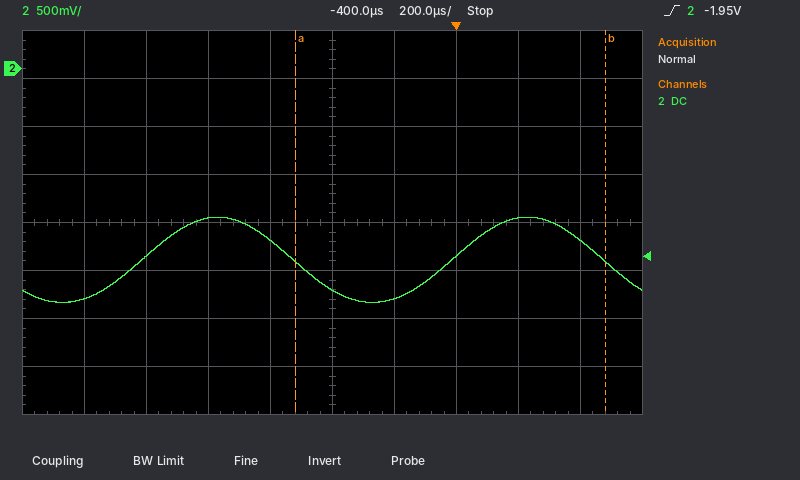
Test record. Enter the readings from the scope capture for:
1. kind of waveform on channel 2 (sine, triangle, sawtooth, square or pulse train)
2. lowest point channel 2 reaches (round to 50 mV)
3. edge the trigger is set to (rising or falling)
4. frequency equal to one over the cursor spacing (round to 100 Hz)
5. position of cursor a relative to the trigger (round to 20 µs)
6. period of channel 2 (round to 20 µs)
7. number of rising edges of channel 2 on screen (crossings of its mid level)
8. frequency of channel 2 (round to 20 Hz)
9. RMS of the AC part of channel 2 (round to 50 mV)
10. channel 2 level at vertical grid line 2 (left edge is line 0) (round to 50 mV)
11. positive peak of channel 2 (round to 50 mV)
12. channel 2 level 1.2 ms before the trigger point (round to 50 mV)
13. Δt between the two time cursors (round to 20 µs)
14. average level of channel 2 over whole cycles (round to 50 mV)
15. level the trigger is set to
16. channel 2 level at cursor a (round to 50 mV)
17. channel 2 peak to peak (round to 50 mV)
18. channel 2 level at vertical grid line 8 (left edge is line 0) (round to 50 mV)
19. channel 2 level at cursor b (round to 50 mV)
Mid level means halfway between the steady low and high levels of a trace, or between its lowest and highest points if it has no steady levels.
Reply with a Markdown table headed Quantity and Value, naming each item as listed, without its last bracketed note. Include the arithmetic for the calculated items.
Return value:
| Quantity | Value |
|---|---|
| kind of waveform on channel 2 | sine |
| lowest point channel 2 reaches | -2.45 V |
| edge the trigger is set to | rising |
| frequency equal to one over the cursor spacing | 1 / 1.00 ms ≈ 1.0 kHz |
| position of cursor a relative to the trigger | -520 µs |
| period of channel 2 | 1.00 ms |
| number of rising edges of channel 2 on screen | 2 |
| frequency of channel 2 | 1 / 1.00 ms ≈ 1.00 kHz |
| RMS of the AC part of channel 2 | 900 mV / (2√2) ≈ 318 mV, so 300 mV to the nearest 50 mV |
| channel 2 level at vertical grid line 2 (left edge is line 0) | -1.95 V |
| positive peak of channel 2 | -1.55 V |
| channel 2 level 1.2 ms before the trigger point | -2.40 V |
| Δt between the two time cursors | 1.00 ms |
| average level of channel 2 over whole cycles | (-1.55 V + (-2.45 V)) / 2 ≈ -2.00 V |
| level the trigger is set to | -1.95 V |
| channel 2 level at cursor a | -2.00 V |
| channel 2 peak to peak | -1.55 V − (-2.45 V) = 900 mV |
| channel 2 level at vertical grid line 8 (left edge is line 0) | -1.55 V |
| channel 2 level at cursor b | -2.00 V |
